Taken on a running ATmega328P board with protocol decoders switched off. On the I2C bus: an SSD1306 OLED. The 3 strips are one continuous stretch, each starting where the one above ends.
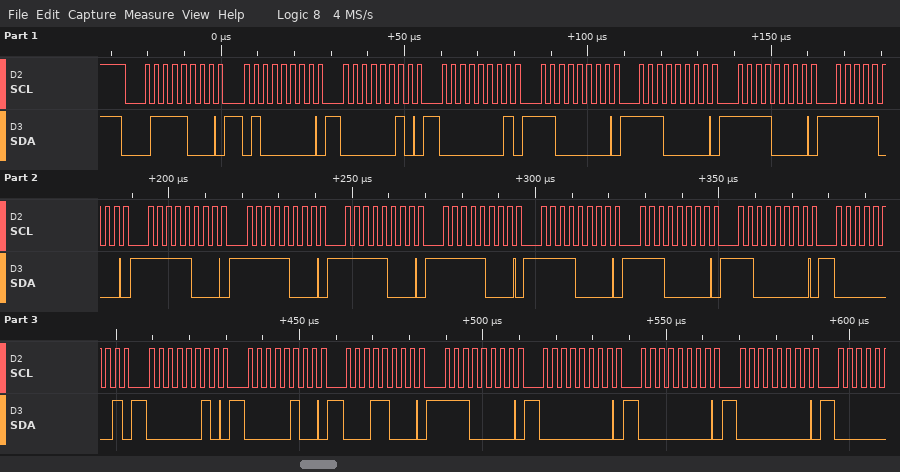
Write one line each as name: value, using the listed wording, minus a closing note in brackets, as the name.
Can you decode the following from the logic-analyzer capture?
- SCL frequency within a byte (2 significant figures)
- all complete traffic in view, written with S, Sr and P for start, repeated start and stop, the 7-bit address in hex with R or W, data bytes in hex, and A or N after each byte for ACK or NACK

SCL frequency within a byte: 400 kHz
all complete traffic in view, written with S, Sr and P for start, repeated start and stop, the 7-bit address in hex with R or W, data bytes in hex, and A or N after each byte for ACK or NACK: S 3CW A 40 A 02 A 01 A C0 A E0 A F0 A F8 A F8 A F8 A F8 A F8 A F0 A E0 A C0 A 01 A 02 A 04 A 18 A E0 A 00 A 00 A 00 A
